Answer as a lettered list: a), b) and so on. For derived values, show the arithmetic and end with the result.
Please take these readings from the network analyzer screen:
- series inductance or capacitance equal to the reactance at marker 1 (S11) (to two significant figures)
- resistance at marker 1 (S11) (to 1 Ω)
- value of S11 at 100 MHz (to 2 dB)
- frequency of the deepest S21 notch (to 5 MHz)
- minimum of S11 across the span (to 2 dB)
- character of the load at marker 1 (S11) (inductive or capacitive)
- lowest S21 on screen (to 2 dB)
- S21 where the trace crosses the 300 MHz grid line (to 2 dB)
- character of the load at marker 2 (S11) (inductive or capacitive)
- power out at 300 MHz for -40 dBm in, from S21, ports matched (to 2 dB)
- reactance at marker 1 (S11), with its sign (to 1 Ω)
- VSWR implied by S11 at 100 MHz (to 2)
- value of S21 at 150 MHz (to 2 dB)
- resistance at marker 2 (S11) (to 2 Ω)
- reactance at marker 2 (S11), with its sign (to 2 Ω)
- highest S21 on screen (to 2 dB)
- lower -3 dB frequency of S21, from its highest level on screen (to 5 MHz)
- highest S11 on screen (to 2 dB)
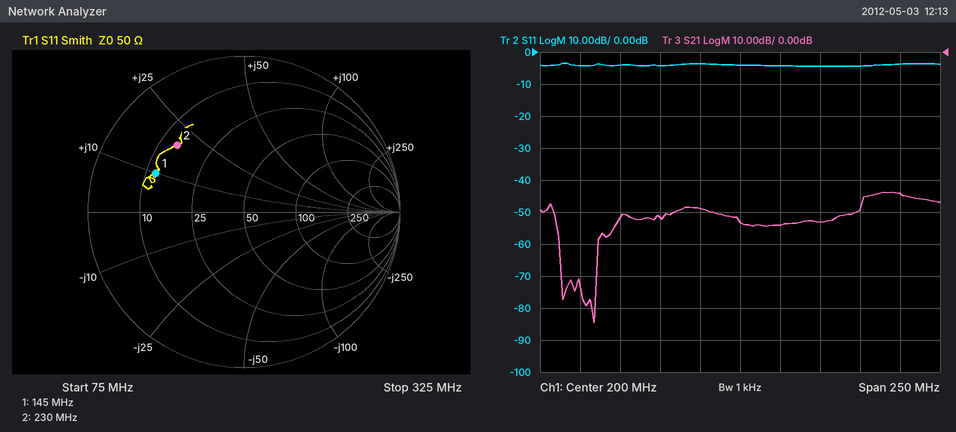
a) L = 10 Ω/(2π × 145 MHz) ≈ 11 nH
b) 12 Ω
c) -4 dB
d) 110 MHz
e) -4 dB
f) inductive
g) -84 dB
h) -44 dB
i) inductive
j) -40 dBm + (-44 dB) = -84 dBm
k) +10 Ω
l) |Γ| = 10^(-4/20) = 0.6310; VSWR = (1 + 0.6310)/(1 − 0.6310) ≈ 4
m) -52 dB
n) 14 Ω
o) +20 Ω
p) -44 dB
q) 275 MHz
r) -4 dB
